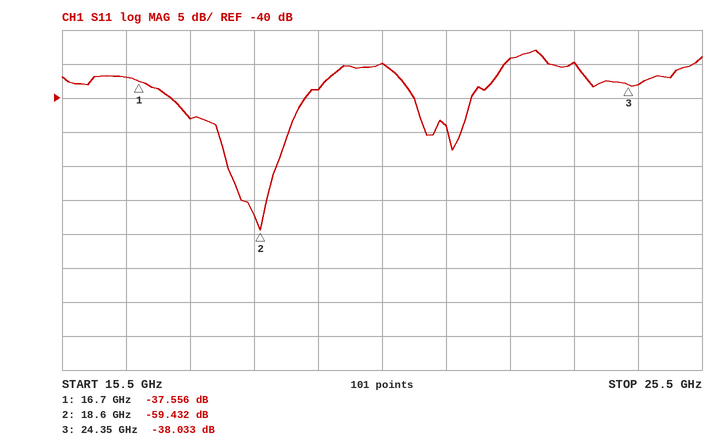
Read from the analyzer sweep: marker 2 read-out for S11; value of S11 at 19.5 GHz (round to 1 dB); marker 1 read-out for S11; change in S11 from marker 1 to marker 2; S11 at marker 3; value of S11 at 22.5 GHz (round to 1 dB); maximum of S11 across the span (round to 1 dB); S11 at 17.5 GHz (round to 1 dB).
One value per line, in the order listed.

-59.432 dB
-39 dB
-37.556 dB
-21.876 dB
-38.033 dB
-34 dB
-33 dB
-43 dB
